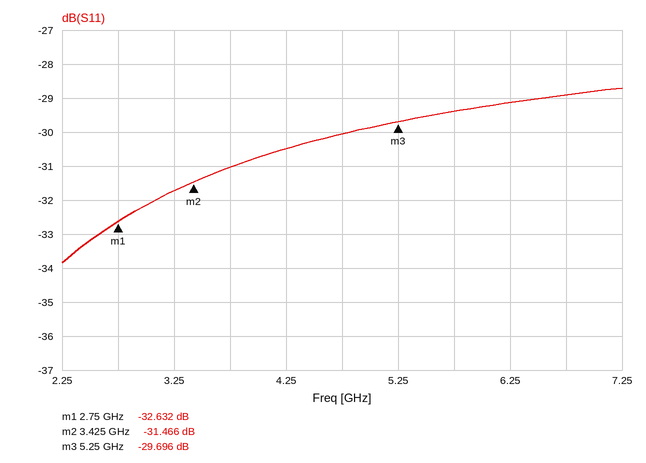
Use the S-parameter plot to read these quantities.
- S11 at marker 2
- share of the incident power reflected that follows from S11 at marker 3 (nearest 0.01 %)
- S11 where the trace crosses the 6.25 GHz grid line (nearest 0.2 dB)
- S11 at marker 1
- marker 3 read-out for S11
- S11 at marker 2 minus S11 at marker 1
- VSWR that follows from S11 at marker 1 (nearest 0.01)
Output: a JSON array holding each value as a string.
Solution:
["-31.466 dB", "0.11 %", "-29.2 dB", "-32.632 dB", "-29.696 dB", "1.166 dB", "1.05"]
